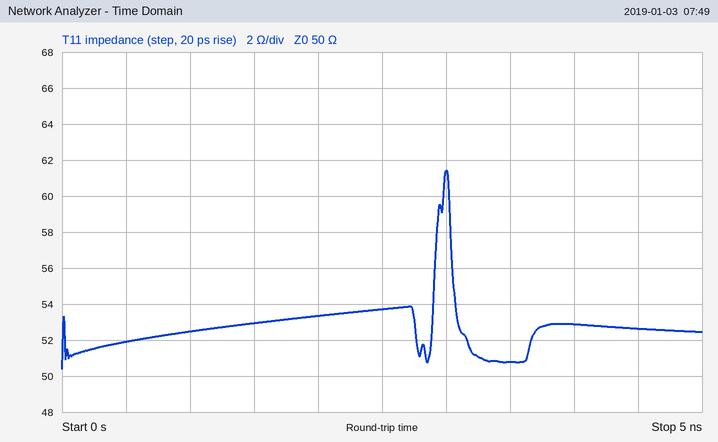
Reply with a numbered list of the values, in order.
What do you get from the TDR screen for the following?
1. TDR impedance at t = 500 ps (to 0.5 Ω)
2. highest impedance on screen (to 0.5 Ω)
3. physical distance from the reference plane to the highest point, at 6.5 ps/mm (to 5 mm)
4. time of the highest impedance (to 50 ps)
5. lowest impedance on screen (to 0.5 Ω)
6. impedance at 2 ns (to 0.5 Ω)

1. 52.0 Ω
2. 61.5 Ω
3. 230 mm
4. 3.00 ns
5. 50.5 Ω
6. 53.5 Ω
